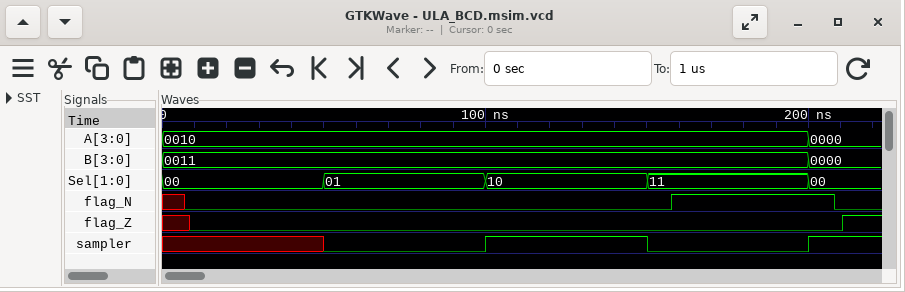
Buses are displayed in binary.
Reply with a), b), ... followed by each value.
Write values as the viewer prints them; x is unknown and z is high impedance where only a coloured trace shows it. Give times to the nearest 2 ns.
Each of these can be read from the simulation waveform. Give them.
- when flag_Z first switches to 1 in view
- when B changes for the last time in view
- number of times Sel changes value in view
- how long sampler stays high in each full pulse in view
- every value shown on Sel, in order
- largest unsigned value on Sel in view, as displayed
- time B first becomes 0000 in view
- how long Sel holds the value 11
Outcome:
a) 210 ns
b) 200 ns
c) 4
d) 50 ns
e) 00, 01, 10, 11, 00
f) 11
g) 200 ns
h) 50 ns
